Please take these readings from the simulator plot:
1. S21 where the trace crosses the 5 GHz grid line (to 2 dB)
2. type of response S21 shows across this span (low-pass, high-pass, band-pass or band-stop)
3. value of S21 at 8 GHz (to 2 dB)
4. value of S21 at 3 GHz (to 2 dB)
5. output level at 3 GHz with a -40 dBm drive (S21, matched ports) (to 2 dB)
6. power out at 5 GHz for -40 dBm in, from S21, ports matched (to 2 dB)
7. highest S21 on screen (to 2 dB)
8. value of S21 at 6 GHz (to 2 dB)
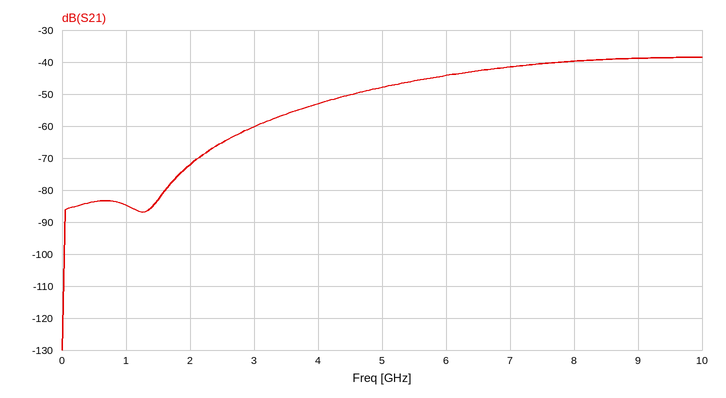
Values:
-48 dB
high-pass
-40 dB
-60 dB
-100 dBm
-88 dBm
-38 dB
-44 dB
